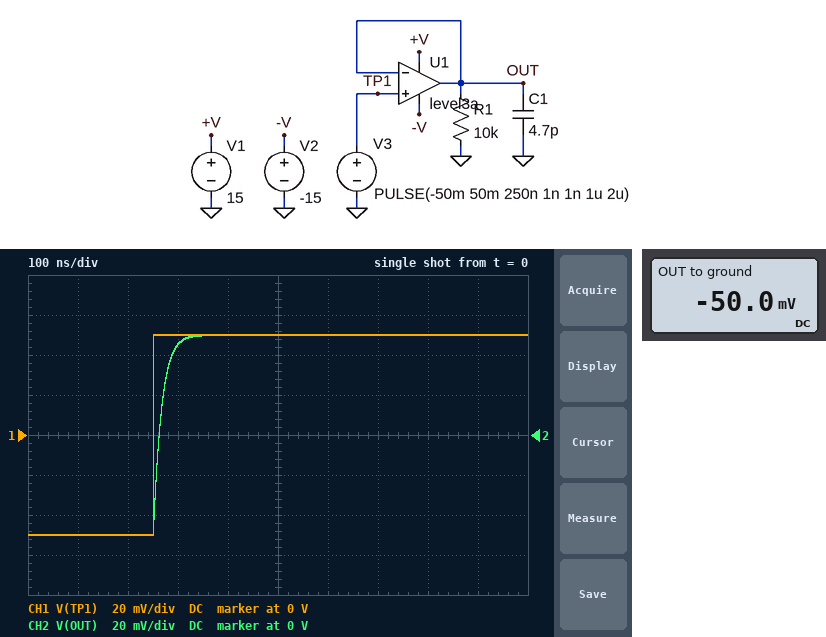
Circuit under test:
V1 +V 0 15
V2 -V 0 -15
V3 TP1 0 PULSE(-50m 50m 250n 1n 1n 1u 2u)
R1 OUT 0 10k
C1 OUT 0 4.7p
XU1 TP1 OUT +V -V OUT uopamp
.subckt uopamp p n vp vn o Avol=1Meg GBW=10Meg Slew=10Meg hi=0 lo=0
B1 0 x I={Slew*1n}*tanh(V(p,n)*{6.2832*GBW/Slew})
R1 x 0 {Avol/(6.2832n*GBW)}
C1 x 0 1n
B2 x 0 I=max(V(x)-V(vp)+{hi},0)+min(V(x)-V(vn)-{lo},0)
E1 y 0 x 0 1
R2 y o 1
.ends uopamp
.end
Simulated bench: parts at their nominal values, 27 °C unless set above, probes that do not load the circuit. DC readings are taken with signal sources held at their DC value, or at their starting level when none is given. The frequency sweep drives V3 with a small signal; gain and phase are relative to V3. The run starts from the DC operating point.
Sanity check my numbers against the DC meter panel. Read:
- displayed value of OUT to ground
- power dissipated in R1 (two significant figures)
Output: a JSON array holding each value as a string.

["-50.0 mV", "250 nW"]
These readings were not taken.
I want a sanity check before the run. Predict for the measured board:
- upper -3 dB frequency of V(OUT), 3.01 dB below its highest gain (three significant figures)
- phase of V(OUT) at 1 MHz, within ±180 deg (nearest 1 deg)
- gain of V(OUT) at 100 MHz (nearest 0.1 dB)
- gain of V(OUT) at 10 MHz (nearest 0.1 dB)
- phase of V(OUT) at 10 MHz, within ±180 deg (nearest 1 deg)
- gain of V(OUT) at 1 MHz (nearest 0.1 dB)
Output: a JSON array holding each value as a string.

["10.0 MHz", "-6 deg", "-20.0 dB", "-3.0 dB", "-45 deg", "0 dB"]
